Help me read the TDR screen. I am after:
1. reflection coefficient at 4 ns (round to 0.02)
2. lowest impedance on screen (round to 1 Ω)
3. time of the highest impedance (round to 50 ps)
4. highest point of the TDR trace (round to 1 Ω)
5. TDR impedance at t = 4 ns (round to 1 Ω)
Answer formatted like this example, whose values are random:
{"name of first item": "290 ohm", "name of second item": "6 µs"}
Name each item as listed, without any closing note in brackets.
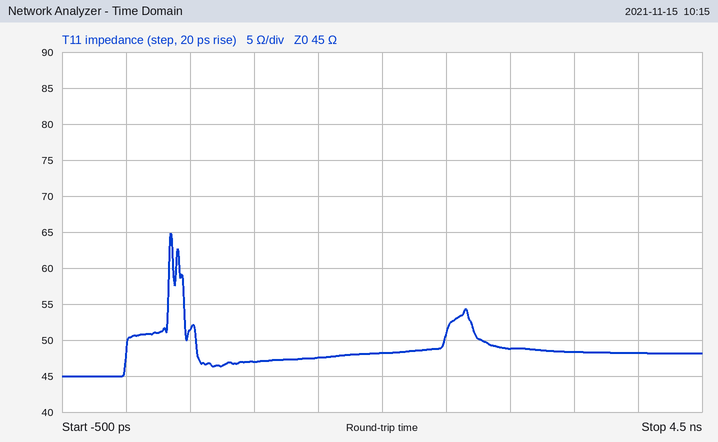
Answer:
{"reflection coefficient at 4 ns": "+0.04", "lowest impedance on screen": "45 Ω", "time of the highest impedance": "350 ps", "highest point of the TDR trace": "65 Ω", "TDR impedance at t = 4 ns": "48 Ω"}
